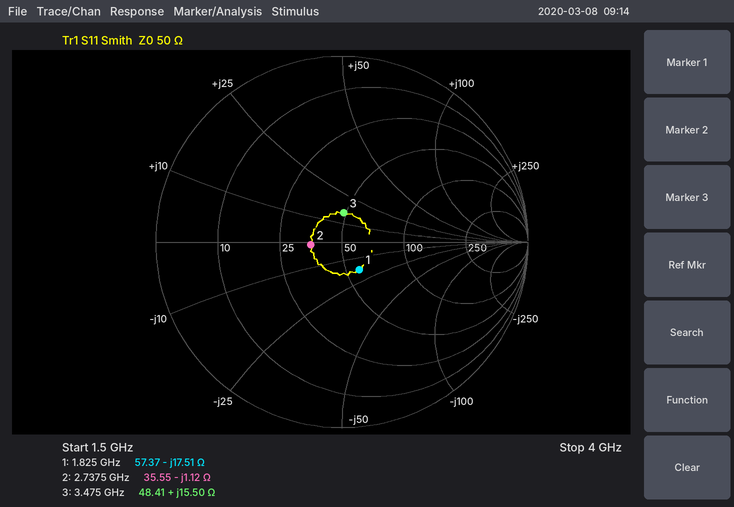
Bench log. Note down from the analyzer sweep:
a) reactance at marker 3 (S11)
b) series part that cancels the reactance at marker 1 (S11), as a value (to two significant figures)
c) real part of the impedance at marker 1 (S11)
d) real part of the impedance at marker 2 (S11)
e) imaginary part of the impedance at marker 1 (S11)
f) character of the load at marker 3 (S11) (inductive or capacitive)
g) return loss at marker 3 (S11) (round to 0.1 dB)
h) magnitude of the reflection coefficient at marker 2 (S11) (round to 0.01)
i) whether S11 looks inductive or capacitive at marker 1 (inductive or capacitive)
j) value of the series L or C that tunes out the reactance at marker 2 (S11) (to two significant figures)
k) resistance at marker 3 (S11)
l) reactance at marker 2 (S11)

+15.50 Ω
1.5 nH
57.37 Ω
35.55 Ω
-17.51 Ω
inductive
16.1 dB
0.17
capacitive
65 pH
48.41 Ω
-1.12 Ω
